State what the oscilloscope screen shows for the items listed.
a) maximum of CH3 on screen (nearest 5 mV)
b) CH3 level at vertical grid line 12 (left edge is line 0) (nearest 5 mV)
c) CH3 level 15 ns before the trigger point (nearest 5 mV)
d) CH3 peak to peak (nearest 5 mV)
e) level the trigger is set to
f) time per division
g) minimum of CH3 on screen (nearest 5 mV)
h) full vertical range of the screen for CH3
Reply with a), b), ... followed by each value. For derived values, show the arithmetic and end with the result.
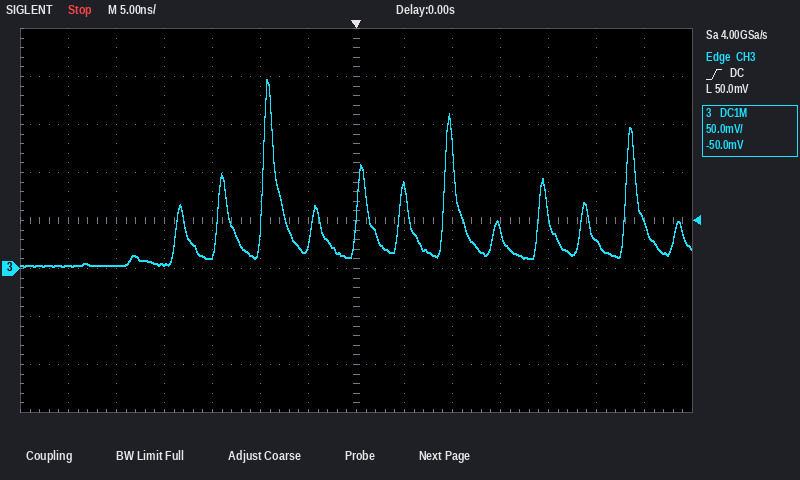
a) 195 mV
b) 30 mV
c) 15 mV
d) 195 mV − (0 mV) = 195 mV
e) 50.0 mV
f) 5 ns
g) 0 mV
h) 400 mV
